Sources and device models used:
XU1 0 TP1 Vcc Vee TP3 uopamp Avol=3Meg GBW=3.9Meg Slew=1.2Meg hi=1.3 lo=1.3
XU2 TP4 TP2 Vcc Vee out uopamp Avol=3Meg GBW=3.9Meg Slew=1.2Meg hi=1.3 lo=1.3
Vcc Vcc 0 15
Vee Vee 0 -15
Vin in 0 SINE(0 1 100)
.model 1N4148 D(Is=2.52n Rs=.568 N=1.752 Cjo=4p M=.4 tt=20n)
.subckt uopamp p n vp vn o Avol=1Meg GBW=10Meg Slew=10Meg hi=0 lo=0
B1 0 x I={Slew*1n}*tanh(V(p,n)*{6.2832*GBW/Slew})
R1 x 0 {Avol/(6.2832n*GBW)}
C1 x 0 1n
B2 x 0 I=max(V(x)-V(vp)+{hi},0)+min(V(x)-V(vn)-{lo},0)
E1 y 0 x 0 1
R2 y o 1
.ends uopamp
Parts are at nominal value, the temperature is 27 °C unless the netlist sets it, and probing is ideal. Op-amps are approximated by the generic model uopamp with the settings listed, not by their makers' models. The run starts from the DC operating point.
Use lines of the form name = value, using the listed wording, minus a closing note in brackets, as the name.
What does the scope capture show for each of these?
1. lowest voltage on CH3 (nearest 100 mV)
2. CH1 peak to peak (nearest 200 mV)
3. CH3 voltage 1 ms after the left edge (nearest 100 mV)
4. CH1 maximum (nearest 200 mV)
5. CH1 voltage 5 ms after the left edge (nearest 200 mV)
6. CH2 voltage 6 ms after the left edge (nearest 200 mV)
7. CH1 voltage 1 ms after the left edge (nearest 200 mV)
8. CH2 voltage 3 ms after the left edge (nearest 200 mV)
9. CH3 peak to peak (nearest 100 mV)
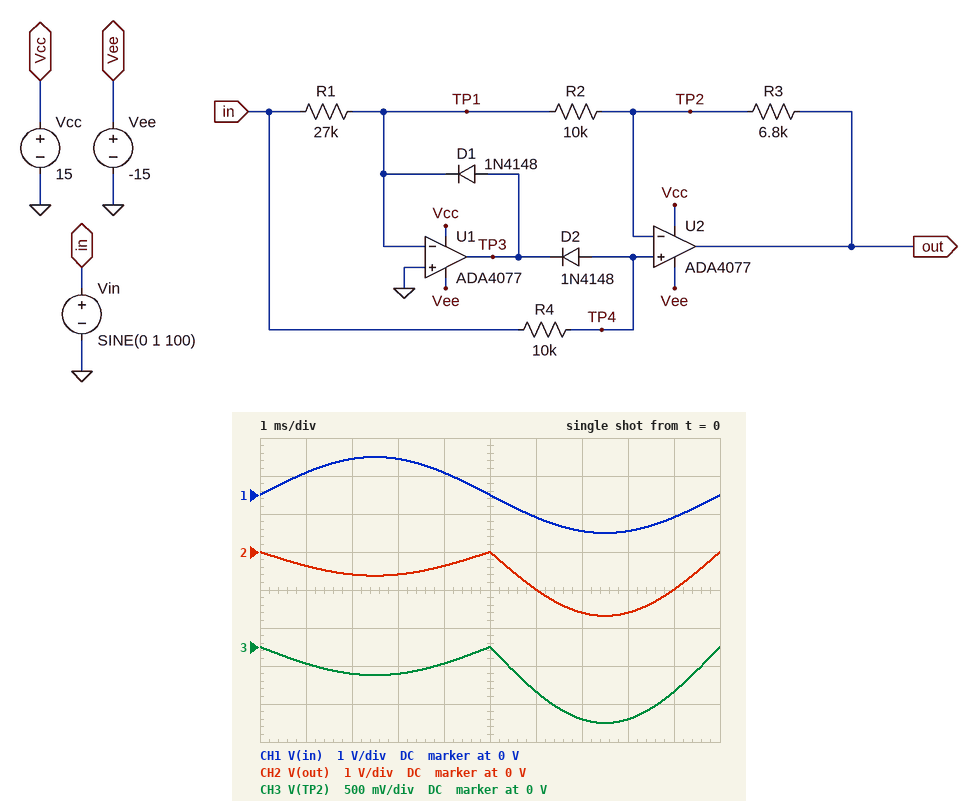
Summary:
lowest voltage on CH3 = -1.0 V
CH1 peak to peak = 2.0 V
CH3 voltage 1 ms after the left edge = -200 mV
CH1 maximum = 1.0 V
CH1 voltage 5 ms after the left edge = 0 V
CH2 voltage 6 ms after the left edge = -1.0 V
CH1 voltage 1 ms after the left edge = 600 mV
CH2 voltage 3 ms after the left edge = -600 mV
CH3 peak to peak = 1.0 V
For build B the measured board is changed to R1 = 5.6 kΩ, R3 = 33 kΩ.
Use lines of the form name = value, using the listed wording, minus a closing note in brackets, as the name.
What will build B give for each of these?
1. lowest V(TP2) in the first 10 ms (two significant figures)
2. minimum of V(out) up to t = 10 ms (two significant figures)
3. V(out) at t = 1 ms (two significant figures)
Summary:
lowest V(TP2) in the first 10 ms = -1.8 V
minimum of V(out) up to t = 10 ms = -7.7 V
V(out) at t = 1 ms = -4.5 V
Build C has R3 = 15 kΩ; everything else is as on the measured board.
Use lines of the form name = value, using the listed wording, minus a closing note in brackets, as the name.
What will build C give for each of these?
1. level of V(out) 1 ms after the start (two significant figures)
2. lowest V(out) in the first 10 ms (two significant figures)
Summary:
level of V(out) 1 ms after the start = -540 mV
lowest V(out) in the first 10 ms = -2.5 V
